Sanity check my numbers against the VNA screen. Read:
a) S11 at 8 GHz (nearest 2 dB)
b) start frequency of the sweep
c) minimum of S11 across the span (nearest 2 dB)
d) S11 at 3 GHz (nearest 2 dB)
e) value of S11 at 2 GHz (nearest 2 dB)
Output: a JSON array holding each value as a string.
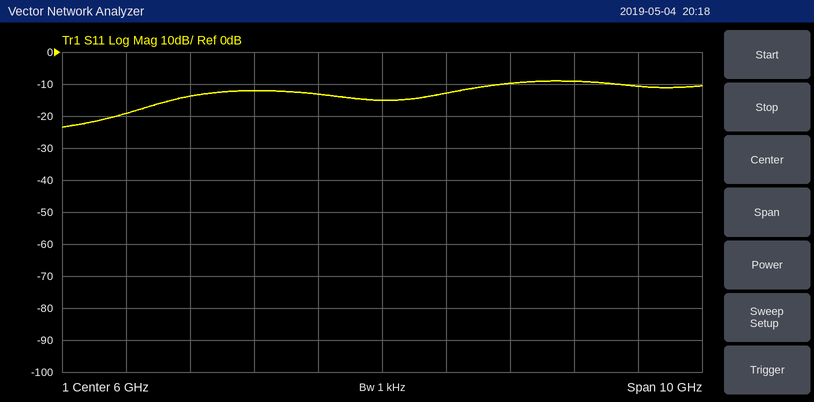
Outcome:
["-10 dB", "1 GHz", "-24 dB", "-14 dB", "-20 dB"]
